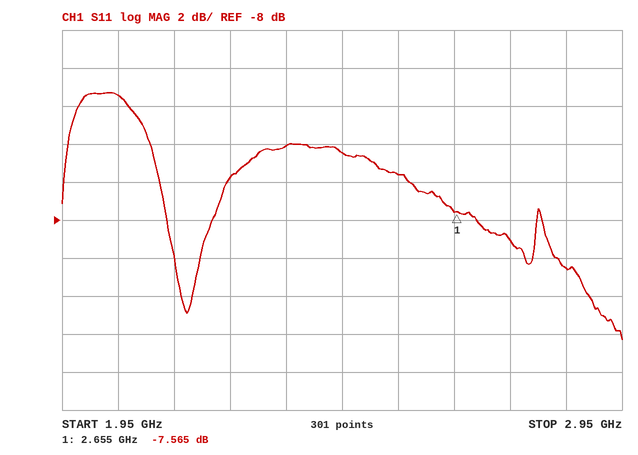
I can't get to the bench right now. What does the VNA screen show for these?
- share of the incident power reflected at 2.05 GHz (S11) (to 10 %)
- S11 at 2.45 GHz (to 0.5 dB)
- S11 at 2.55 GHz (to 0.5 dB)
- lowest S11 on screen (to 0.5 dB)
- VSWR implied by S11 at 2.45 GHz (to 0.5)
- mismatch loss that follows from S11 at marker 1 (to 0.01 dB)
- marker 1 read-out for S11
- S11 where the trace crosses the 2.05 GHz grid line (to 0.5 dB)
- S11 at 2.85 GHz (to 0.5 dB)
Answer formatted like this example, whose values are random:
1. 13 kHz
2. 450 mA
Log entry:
1. 70 %
2. -4.5 dB
3. -5.5 dB
4. -14.5 dB
5. 4.0
6. 0.84 dB
7. -7.565 dB
8. -1.5 dB
9. -10.5 dB
